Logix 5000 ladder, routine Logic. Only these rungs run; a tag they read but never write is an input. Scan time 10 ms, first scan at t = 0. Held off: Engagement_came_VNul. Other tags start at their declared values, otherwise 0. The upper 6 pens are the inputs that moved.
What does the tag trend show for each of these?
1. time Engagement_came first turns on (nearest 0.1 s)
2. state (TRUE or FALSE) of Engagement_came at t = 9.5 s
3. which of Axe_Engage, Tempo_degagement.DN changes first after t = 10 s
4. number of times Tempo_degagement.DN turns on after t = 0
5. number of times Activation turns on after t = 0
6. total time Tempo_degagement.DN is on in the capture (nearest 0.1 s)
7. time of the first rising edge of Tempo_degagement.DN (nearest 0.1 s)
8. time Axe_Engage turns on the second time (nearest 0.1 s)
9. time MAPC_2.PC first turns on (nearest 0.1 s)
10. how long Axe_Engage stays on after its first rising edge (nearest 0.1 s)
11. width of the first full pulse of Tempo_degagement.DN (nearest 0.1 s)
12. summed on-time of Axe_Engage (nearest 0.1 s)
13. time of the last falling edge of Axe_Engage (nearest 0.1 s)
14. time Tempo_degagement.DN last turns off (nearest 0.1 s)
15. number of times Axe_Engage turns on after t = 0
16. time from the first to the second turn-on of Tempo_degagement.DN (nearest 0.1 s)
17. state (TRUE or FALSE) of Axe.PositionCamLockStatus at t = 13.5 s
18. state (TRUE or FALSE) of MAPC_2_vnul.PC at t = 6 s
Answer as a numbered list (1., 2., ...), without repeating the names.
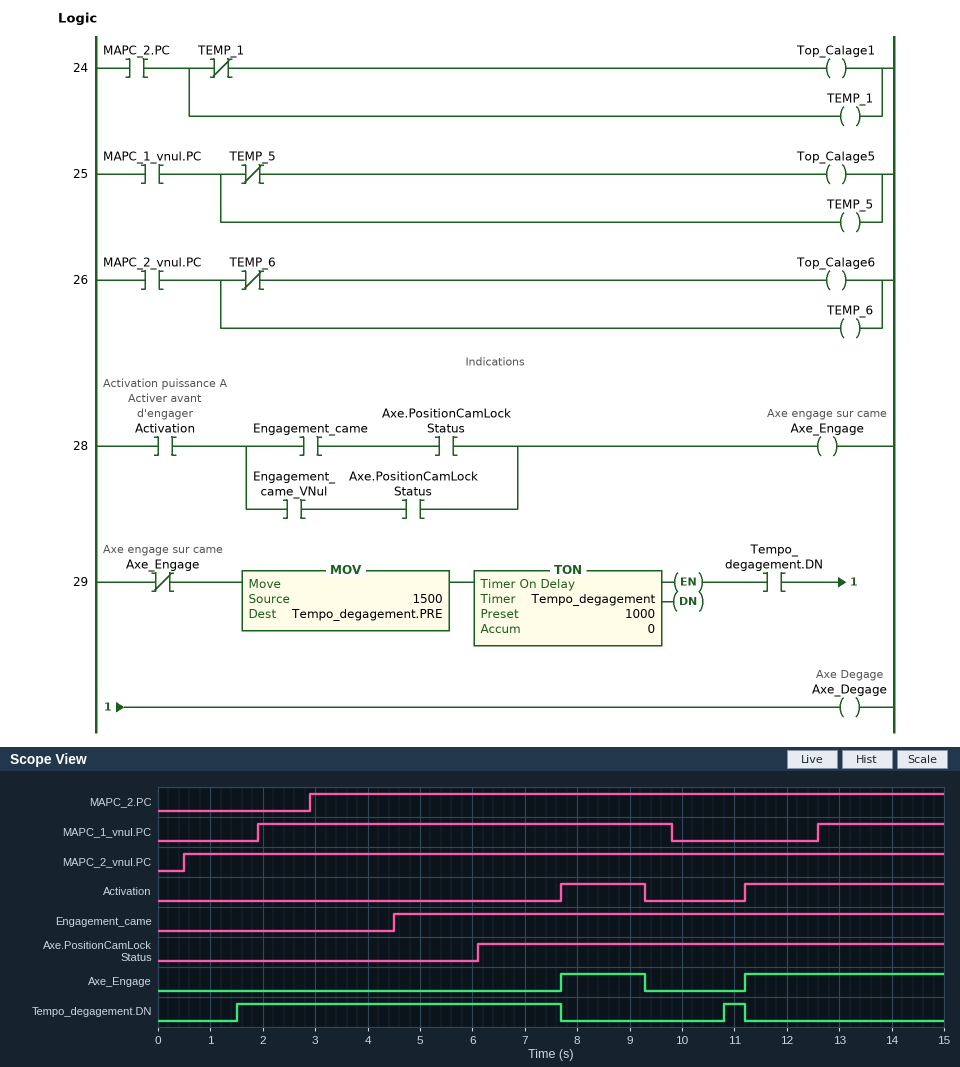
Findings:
1. 4.5 s
2. TRUE
3. Tempo_degagement.DN
4. 2
5. 2
6. 6.6 s
7. 1.5 s
8. 11.2 s
9. 2.9 s
10. 1.6 s
11. 6.2 s
12. 5.4 s
13. 9.3 s
14. 11.2 s
15. 2
16. 9.3 s
17. TRUE
18. TRUE
